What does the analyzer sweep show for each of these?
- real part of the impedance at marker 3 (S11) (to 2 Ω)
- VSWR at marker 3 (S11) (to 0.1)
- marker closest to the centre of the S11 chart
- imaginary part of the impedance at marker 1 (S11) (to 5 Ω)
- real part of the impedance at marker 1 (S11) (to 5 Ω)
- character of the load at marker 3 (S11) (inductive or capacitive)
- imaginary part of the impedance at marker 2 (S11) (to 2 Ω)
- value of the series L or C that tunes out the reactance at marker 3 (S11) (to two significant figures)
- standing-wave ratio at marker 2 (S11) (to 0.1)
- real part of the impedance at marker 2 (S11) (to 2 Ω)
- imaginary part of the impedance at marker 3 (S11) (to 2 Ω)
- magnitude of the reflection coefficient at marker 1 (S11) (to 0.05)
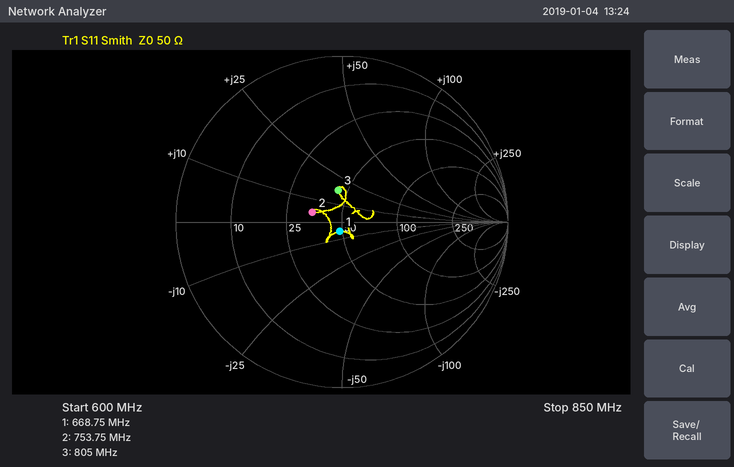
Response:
44 Ω
1.5
marker 1
-5 Ω
50 Ω
inductive
+4 Ω
11 pF
1.5
34 Ω
+18 Ω
0.05
